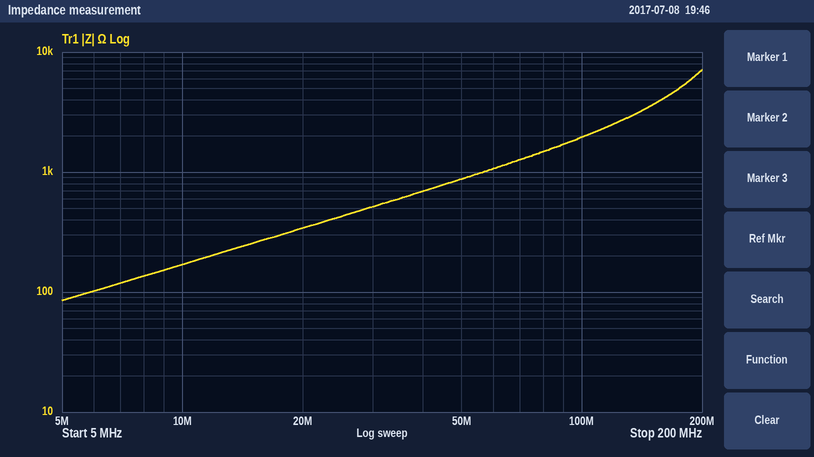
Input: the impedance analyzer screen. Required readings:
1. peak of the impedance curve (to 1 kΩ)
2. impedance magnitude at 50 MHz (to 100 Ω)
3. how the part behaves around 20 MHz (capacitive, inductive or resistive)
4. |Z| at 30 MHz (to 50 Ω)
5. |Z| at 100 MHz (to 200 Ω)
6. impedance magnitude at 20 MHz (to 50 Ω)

7 kΩ
900 Ω
inductive
500 Ω
2.0 kΩ
350 Ω
